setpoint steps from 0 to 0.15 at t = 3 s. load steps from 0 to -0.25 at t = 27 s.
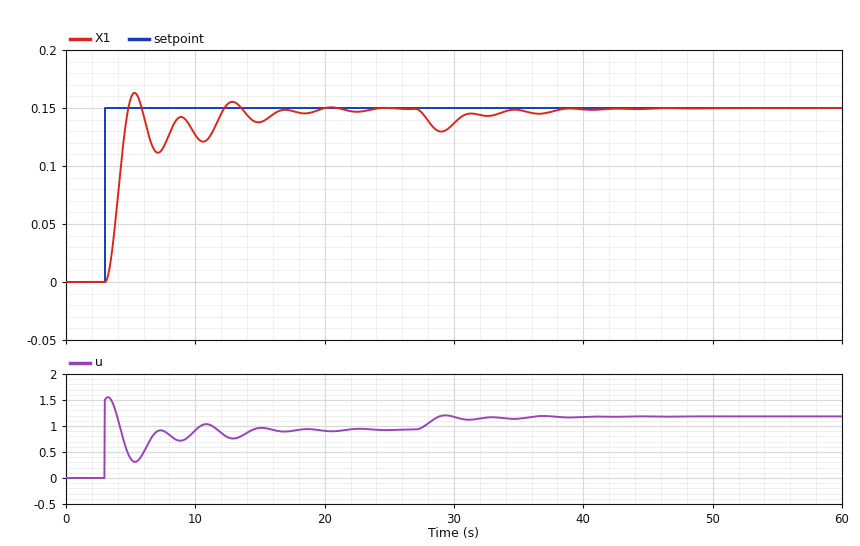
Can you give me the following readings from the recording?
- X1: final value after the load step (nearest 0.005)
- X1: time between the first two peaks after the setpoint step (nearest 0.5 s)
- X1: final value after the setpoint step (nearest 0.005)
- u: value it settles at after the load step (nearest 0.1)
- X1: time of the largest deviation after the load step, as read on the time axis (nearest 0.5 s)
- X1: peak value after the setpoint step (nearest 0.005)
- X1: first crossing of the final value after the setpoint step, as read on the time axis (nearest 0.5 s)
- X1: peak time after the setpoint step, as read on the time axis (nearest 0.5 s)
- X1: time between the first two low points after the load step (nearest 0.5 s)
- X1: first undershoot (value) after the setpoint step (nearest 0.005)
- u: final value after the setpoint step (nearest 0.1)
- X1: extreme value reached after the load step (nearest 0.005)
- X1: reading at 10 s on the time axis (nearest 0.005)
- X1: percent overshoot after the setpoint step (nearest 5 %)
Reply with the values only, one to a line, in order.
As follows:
0.150
3.5 s
0.150
1.2
29.0 s
0.165
5.0 s
5.5 s
3.5 s
0.110
0.9
0.130
0.125
10 %
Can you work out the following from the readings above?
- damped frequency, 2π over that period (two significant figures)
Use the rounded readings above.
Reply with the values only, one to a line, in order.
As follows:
1.8 rad/s
